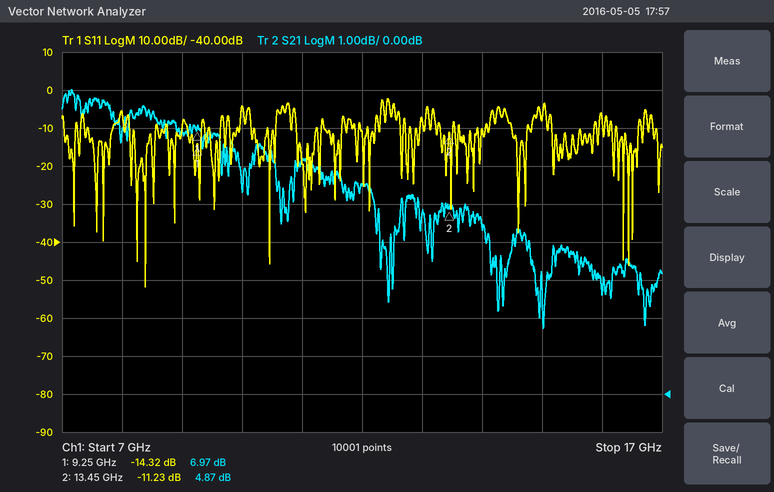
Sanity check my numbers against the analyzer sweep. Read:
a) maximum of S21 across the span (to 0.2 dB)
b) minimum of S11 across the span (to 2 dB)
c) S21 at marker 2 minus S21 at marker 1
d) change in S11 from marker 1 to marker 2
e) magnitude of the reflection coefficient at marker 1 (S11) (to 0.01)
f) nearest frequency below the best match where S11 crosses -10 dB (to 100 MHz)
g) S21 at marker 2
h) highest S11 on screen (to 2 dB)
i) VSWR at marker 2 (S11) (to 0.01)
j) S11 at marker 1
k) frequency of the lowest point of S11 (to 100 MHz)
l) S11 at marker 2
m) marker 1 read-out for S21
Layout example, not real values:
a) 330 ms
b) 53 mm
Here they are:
a) 8.0 dB
b) -52 dB
c) -2.10 dB
d) 3.09 dB
e) 0.19
f) 8.1 GHz
g) 4.87 dB
h) -2 dB
i) 1.76
j) -14.32 dB
k) 8.4 GHz
l) -11.23 dB
m) 6.97 dB
